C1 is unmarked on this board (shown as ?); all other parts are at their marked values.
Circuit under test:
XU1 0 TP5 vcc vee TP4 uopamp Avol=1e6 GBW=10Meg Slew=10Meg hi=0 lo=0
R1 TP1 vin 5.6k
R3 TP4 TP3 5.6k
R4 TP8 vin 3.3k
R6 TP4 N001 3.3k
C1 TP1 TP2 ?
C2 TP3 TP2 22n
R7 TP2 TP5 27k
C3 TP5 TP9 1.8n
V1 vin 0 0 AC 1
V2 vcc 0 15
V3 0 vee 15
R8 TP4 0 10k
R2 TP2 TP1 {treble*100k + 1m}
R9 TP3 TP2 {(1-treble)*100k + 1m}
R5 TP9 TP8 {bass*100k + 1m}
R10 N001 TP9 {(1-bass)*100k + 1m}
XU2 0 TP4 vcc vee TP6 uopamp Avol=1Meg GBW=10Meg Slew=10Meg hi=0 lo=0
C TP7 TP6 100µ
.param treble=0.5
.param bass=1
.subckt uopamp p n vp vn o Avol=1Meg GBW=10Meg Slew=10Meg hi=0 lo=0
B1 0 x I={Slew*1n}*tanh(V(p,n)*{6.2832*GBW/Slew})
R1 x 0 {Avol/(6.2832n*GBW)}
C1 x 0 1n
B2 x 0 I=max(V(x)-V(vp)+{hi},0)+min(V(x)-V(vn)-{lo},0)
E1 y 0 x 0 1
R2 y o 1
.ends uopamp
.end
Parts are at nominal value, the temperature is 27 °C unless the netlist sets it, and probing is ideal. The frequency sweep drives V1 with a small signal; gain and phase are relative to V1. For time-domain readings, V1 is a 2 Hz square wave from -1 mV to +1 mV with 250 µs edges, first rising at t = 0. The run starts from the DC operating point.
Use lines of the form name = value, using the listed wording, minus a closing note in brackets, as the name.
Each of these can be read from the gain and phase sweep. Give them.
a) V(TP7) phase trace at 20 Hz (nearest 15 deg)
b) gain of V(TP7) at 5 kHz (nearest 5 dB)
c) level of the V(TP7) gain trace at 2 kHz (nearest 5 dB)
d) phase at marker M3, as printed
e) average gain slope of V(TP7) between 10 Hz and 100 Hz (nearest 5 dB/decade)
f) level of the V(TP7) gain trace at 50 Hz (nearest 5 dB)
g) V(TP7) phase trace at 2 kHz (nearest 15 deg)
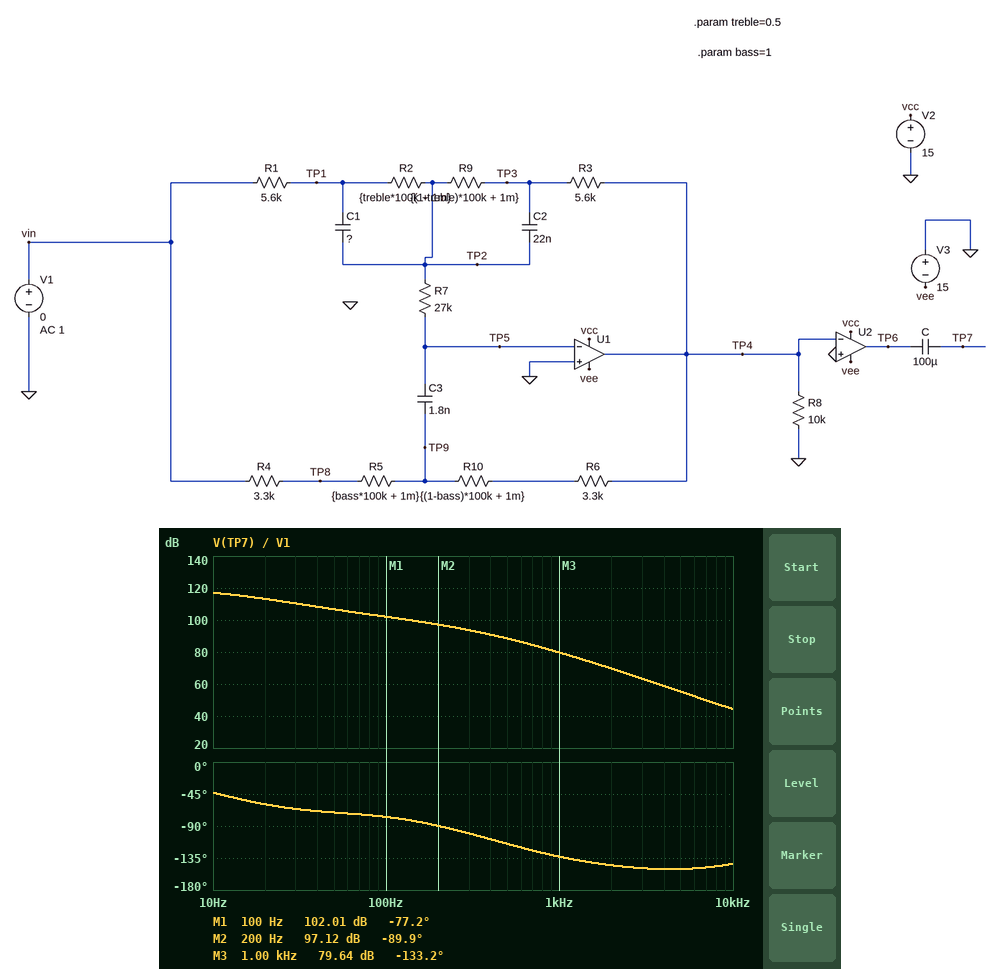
V(TP7) phase trace at 20 Hz = -60 deg
gain of V(TP7) at 5 kHz = 55 dB
level of the V(TP7) gain trace at 2 kHz = 70 dB
phase at marker M3, as printed = -133.2 deg
average gain slope of V(TP7) between 10 Hz and 100 Hz = -15 dB/decade
level of the V(TP7) gain trace at 50 Hz = 105 dB
V(TP7) phase trace at 2 kHz = -150 deg
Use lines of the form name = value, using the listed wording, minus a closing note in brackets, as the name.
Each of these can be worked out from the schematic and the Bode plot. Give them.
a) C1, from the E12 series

C1, from the E12 series = 39 nF
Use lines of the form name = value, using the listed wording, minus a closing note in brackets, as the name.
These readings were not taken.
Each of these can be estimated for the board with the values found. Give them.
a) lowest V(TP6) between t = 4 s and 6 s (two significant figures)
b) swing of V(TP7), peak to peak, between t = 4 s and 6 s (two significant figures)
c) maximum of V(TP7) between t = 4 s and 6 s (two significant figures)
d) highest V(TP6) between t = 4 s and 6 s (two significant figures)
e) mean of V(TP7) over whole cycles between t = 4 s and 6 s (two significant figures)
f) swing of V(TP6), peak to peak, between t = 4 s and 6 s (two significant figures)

lowest V(TP6) between t = 4 s and 6 s = -15 V
swing of V(TP7), peak to peak, between t = 4 s and 6 s = 30 V
maximum of V(TP7) between t = 4 s and 6 s = 30 V
highest V(TP6) between t = 4 s and 6 s = 15 V
mean of V(TP7) over whole cycles between t = 4 s and 6 s = 15 V
swing of V(TP6), peak to peak, between t = 4 s and 6 s = 30 V
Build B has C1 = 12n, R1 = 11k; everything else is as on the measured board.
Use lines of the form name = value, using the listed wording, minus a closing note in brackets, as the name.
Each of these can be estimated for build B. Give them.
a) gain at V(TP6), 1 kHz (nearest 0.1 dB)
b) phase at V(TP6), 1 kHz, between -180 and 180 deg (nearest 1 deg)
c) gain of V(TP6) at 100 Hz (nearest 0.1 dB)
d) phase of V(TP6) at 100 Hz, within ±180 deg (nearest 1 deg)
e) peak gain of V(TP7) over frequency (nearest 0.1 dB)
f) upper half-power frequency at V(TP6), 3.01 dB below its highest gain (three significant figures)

gain at V(TP6), 1 kHz = 72.5 dB
phase at V(TP6), 1 kHz, between -180 and 180 deg = -118 deg
gain of V(TP6) at 100 Hz = 97.7 dB
phase of V(TP6) at 100 Hz, within ±180 deg = -103 deg
peak gain of V(TP7) over frequency = 119.2 dB
upper half-power frequency at V(TP6), 3.01 dB below its highest gain = 9.96 Hz
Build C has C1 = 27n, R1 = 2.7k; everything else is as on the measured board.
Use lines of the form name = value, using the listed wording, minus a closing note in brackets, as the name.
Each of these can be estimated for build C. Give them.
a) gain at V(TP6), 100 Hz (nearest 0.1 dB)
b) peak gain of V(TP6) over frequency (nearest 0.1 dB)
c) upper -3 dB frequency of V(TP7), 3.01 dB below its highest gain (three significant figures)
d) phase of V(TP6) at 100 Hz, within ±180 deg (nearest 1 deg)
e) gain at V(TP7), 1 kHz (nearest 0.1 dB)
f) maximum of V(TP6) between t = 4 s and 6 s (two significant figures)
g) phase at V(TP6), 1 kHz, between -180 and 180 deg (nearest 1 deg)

gain at V(TP6), 100 Hz = 100.9 dB
peak gain of V(TP6) over frequency = 120.5 dB
upper -3 dB frequency of V(TP7), 3.01 dB below its highest gain = 10.0 Hz
phase of V(TP6) at 100 Hz, within ±180 deg = -83 deg
gain at V(TP7), 1 kHz = 81.1 dB
maximum of V(TP6) between t = 4 s and 6 s = 15 V
phase at V(TP6), 1 kHz, between -180 and 180 deg = -113 deg
